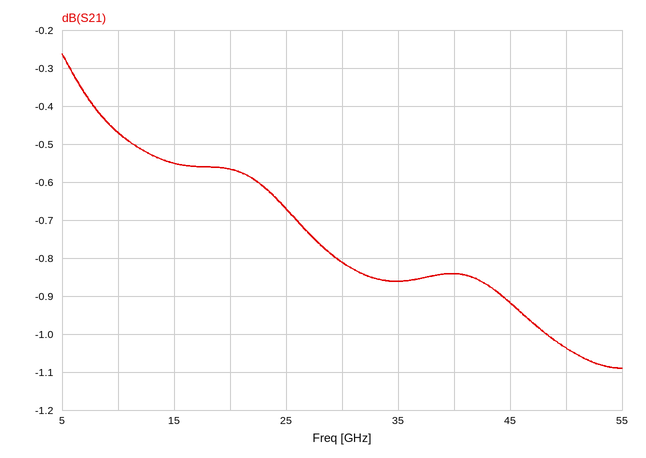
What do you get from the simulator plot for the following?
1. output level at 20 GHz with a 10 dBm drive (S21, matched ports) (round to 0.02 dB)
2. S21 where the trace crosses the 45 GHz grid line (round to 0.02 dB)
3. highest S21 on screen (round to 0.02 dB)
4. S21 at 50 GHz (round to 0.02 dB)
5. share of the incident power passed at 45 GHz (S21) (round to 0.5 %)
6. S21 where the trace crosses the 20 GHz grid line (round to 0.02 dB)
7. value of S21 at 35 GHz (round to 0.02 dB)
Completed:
9.44 dBm
-0.92 dB
-0.26 dB
-1.04 dB
81.0 %
-0.56 dB
-0.86 dB
